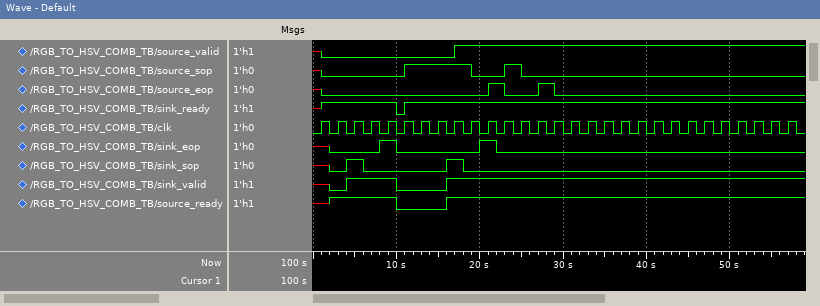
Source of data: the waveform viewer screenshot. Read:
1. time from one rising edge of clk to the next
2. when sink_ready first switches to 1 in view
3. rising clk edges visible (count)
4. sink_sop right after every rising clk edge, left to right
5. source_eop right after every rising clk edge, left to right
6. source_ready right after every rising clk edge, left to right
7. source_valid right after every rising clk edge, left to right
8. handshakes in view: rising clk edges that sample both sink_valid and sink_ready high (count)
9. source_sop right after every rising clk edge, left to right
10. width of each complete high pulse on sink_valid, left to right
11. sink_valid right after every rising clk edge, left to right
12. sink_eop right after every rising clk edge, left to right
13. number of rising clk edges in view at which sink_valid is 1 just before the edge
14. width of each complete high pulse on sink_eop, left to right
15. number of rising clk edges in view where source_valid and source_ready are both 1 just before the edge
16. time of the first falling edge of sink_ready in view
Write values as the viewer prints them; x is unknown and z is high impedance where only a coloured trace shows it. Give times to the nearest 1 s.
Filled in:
2 s
1 s
29
x 0 1 0 0 0 0 0 1 0 0 0 0 0 0 0 0 0 0 0 0 0 0 0 0 0 0 0 0
0 0 0 0 0 0 0 0 0 0 1 0 0 1 0 0 0 0 0 0 0 0 0 0 0 0 0 0 0
x 1 1 1 1 0 0 0 1 1 1 1 1 1 1 1 1 1 1 1 1 1 1 1 1 1 1 1 1
0 0 0 0 0 0 0 0 1 1 1 1 1 1 1 1 1 1 1 1 1 1 1 1 1 1 1 1 1
24
0 0 0 0 0 1 1 1 1 0 0 1 0 0 0 0 0 0 0 0 0 0 0 0 0 0 0 0 0
6 s
x 0 1 1 1 0 0 0 1 1 1 1 1 1 1 1 1 1 1 1 1 1 1 1 1 1 1 1 1
x 0 0 0 1 0 0 0 0 0 1 0 0 0 0 0 0 0 0 0 0 0 0 0 0 0 0 0 0
24
2 s, 2 s
20
10 s
